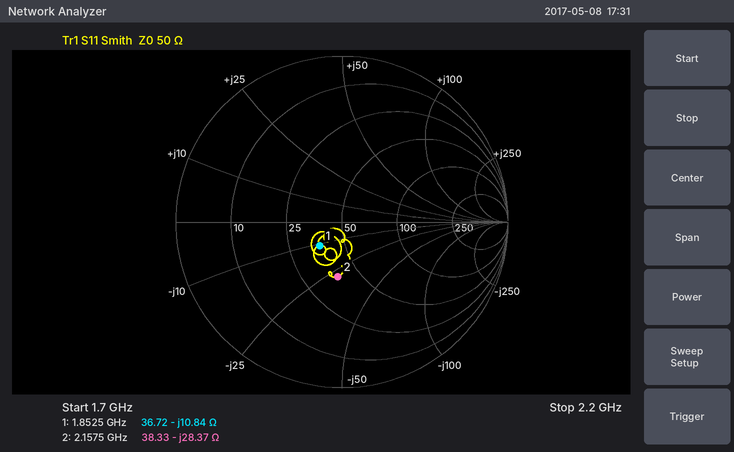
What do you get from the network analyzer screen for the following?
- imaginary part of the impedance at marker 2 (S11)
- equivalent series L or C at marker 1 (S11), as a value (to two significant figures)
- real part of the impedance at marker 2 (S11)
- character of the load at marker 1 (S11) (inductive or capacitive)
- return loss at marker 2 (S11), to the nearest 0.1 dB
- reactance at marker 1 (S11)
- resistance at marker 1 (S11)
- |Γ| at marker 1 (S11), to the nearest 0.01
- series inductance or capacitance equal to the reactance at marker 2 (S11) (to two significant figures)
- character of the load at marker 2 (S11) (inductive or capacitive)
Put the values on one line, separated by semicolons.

-28.37 Ω; 7.9 pF; 38.33 Ω; capacitive; 9.6 dB; -10.84 Ω; 36.72 Ω; 0.20; 2.6 pF; capacitive
